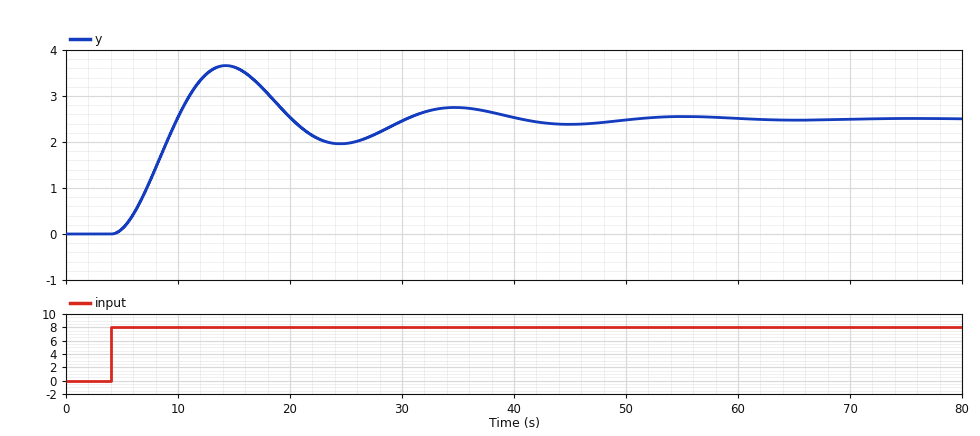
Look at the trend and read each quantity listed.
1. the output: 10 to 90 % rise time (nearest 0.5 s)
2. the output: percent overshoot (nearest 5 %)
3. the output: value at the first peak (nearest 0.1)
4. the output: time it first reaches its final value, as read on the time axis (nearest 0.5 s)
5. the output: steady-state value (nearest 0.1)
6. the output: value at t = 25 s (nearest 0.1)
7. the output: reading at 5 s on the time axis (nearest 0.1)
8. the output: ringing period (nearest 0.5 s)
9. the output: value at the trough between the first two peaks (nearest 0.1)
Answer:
4.0 s
45 %
3.7
10.0 s
2.5
2.0
0.1
20.5 s
2.0
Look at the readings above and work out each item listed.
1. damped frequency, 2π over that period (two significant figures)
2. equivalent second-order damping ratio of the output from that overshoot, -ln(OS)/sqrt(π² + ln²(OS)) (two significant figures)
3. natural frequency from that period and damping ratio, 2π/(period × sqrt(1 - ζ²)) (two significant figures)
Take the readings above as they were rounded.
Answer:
0.31 rad/s
0.25
0.32 rad/s
